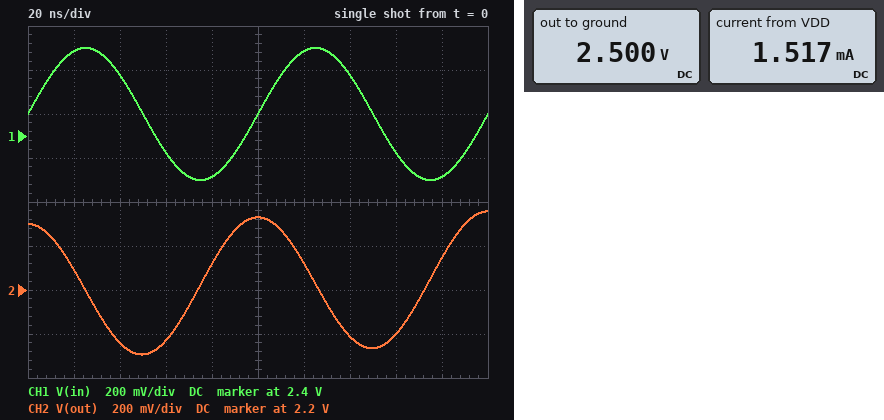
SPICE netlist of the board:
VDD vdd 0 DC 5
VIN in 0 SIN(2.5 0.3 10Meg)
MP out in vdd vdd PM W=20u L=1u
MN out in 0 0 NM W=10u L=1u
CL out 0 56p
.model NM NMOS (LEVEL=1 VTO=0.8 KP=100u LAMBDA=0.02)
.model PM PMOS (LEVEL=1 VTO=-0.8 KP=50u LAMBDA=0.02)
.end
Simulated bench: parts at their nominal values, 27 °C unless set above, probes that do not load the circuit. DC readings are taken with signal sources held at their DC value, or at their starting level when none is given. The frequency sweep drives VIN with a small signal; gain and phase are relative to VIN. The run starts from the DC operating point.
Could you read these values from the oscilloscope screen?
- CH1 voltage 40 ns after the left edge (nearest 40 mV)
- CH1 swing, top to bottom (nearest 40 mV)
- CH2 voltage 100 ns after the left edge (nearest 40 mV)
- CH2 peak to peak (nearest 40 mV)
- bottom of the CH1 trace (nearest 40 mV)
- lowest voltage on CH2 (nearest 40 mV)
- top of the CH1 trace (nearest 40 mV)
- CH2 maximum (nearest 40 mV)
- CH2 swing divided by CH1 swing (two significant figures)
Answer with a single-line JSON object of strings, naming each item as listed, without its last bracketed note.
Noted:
{"CH1 voltage 40 ns after the left edge": "2.68 V", "CH1 swing, top to bottom": "600 mV", "CH2 voltage 100 ns after the left edge": "2.52 V", "CH2 peak to peak": "640 mV", "bottom of the CH1 trace": "2.20 V", "lowest voltage on CH2": "1.92 V", "top of the CH1 trace": "2.80 V", "CH2 maximum": "2.56 V", "CH2 swing divided by CH1 swing": "1.1"}
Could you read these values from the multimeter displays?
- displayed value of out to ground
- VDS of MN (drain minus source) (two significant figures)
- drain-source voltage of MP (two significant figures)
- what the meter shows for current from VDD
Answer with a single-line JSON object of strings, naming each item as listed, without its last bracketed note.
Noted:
{"displayed value of out to ground": "2.500 V", "VDS of MN (drain minus source)": "2.5 V", "drain-source voltage of MP": "-2.5 V", "what the meter shows for current from VDD": "1.517 mA"}
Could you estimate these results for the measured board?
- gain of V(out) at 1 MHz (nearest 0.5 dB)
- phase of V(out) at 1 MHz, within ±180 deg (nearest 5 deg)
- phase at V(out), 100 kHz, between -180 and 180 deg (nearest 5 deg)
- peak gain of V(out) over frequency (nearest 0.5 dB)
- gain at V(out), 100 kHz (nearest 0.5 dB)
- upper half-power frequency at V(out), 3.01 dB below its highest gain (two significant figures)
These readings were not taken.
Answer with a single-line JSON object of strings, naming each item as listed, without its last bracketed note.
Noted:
{"gain of V(out) at 1 MHz": "20.0 dB", "phase of V(out) at 1 MHz, within ±180 deg": "100 deg", "phase at V(out), 100 kHz, between -180 and 180 deg": "150 deg", "peak gain of V(out) over frequency": "36.0 dB", "gain at V(out), 100 kHz": "34.5 dB", "upper half-power frequency at V(out), 3.01 dB below its highest gain": "160 kHz"}
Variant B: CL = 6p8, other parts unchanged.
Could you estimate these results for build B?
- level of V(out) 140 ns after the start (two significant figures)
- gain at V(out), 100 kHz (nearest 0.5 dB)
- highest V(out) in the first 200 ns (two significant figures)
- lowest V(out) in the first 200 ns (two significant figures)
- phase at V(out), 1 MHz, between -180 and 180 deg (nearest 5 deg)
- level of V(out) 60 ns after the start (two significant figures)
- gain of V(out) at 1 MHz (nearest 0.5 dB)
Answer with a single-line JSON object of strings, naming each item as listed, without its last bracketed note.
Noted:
{"level of V(out) 140 ns after the start": "780 mV", "gain at V(out), 100 kHz": "36.0 dB", "highest V(out) in the first 200 ns": "4.2 V", "lowest V(out) in the first 200 ns": "680 mV", "phase at V(out), 1 MHz, between -180 and 180 deg": "145 deg", "level of V(out) 60 ns after the start": "1.7 V", "gain of V(out) at 1 MHz": "34.0 dB"}
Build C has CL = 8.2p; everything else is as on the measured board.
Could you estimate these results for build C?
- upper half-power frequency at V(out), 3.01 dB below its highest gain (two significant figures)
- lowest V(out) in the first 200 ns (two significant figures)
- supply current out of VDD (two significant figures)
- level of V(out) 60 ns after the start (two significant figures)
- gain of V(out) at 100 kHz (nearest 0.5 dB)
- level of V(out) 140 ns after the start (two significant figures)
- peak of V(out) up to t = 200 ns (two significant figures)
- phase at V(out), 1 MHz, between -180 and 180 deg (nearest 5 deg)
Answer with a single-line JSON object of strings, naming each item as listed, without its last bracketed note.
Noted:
{"upper half-power frequency at V(out), 3.01 dB below its highest gain": "1.1 MHz", "lowest V(out) in the first 200 ns": "720 mV", "supply current out of VDD": "1.5 mA", "level of V(out) 60 ns after the start": "1.6 V", "gain of V(out) at 100 kHz": "36.0 dB", "level of V(out) 140 ns after the start": "860 mV", "peak of V(out) up to t = 200 ns": "4.1 V", "phase at V(out), 1 MHz, between -180 and 180 deg": "140 deg"}
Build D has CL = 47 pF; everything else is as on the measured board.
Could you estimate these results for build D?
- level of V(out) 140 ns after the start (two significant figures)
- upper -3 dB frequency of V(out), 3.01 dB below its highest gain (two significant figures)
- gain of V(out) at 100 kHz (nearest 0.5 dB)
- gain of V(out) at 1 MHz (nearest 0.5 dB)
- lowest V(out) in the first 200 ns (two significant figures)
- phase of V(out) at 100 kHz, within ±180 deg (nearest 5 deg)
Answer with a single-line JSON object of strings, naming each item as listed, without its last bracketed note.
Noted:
{"level of V(out) 140 ns after the start": "1.9 V", "upper -3 dB frequency of V(out), 3.01 dB below its highest gain": "200 kHz", "gain of V(out) at 100 kHz": "35.0 dB", "gain of V(out) at 1 MHz": "21.5 dB", "lowest V(out) in the first 200 ns": "1.8 V", "phase of V(out) at 100 kHz, within ±180 deg": "155 deg"}
